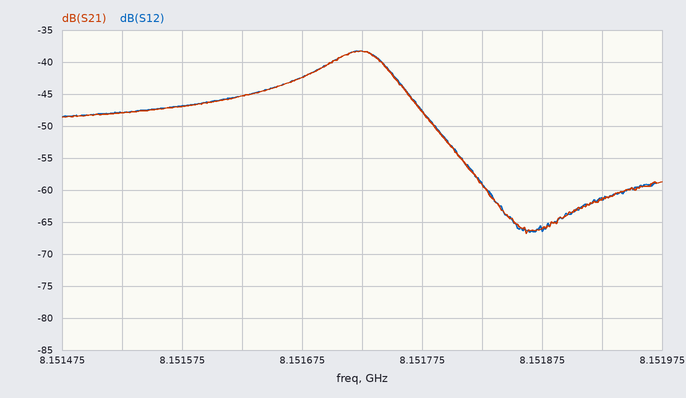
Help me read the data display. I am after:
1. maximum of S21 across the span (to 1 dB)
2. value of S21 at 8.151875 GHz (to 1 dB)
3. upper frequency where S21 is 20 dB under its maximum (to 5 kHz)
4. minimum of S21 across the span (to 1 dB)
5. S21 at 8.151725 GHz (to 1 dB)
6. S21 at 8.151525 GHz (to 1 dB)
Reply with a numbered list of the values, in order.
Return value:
1. -38 dB
2. -66 dB
3. 8.151820 GHz
4. -67 dB
5. -38 dB
6. -48 dB
